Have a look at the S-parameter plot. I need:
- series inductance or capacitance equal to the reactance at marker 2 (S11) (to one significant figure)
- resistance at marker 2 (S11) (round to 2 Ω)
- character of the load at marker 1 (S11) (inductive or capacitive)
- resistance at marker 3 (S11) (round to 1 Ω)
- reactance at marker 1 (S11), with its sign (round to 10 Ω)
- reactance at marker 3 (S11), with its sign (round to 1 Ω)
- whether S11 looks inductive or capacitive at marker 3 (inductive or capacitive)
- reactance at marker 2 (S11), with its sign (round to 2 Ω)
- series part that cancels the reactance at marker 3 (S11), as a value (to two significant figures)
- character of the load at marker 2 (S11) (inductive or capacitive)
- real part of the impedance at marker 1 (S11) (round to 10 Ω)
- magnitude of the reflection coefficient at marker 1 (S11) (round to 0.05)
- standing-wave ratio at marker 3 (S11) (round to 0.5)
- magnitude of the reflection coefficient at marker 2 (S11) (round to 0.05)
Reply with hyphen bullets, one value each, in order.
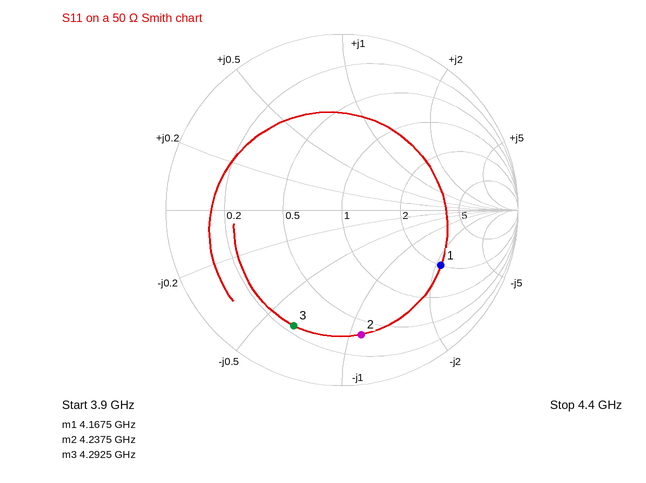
- 700 fF
- 18 Ω
- capacitive
- 12 Ω
- -110 Ω
- -32 Ω
- capacitive
- -54 Ω
- 1.2 nH
- capacitive
- 100 Ω
- 0.65
- 6.0
- 0.70
